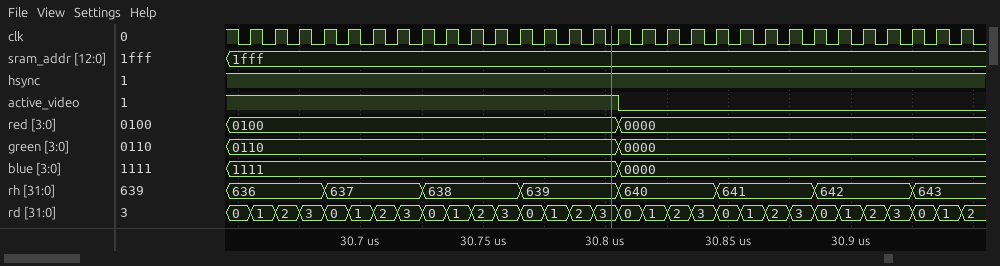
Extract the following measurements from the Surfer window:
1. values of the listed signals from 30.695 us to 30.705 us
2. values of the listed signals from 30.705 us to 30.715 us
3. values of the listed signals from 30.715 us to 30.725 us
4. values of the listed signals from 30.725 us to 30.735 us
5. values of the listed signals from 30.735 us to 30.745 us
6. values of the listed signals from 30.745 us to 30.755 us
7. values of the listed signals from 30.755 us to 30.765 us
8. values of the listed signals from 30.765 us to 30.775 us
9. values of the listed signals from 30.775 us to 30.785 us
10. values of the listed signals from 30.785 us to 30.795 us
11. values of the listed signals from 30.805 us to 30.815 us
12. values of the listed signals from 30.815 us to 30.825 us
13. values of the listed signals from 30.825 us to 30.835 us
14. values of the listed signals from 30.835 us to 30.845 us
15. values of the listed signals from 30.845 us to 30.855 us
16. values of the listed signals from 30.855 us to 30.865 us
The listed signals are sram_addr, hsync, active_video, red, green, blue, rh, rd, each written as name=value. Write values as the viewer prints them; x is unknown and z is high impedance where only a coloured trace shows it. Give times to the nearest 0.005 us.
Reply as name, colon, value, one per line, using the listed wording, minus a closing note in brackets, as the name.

values of the listed signals from 30.695 us to 30.705 us: sram_addr=1fff, hsync=1, active_video=1, red=0100, green=0110, blue=1111, rh=637, rd=1
values of the listed signals from 30.705 us to 30.715 us: sram_addr=1fff, hsync=1, active_video=1, red=0100, green=0110, blue=1111, rh=637, rd=2
values of the listed signals from 30.715 us to 30.725 us: sram_addr=1fff, hsync=1, active_video=1, red=0100, green=0110, blue=1111, rh=637, rd=3
values of the listed signals from 30.725 us to 30.735 us: sram_addr=1fff, hsync=1, active_video=1, red=0100, green=0110, blue=1111, rh=638, rd=0
values of the listed signals from 30.735 us to 30.745 us: sram_addr=1fff, hsync=1, active_video=1, red=0100, green=0110, blue=1111, rh=638, rd=1
values of the listed signals from 30.745 us to 30.755 us: sram_addr=1fff, hsync=1, active_video=1, red=0100, green=0110, blue=1111, rh=638, rd=2
values of the listed signals from 30.755 us to 30.765 us: sram_addr=1fff, hsync=1, active_video=1, red=0100, green=0110, blue=1111, rh=638, rd=3
values of the listed signals from 30.765 us to 30.775 us: sram_addr=1fff, hsync=1, active_video=1, red=0100, green=0110, blue=1111, rh=639, rd=0
values of the listed signals from 30.775 us to 30.785 us: sram_addr=1fff, hsync=1, active_video=1, red=0100, green=0110, blue=1111, rh=639, rd=1
values of the listed signals from 30.785 us to 30.795 us: sram_addr=1fff, hsync=1, active_video=1, red=0100, green=0110, blue=1111, rh=639, rd=2
values of the listed signals from 30.805 us to 30.815 us: sram_addr=1fff, hsync=1, active_video=0, red=0000, green=0000, blue=0000, rh=640, rd=0
values of the listed signals from 30.815 us to 30.825 us: sram_addr=1fff, hsync=1, active_video=0, red=0000, green=0000, blue=0000, rh=640, rd=1
values of the listed signals from 30.825 us to 30.835 us: sram_addr=1fff, hsync=1, active_video=0, red=0000, green=0000, blue=0000, rh=640, rd=2
values of the listed signals from 30.835 us to 30.845 us: sram_addr=1fff, hsync=1, active_video=0, red=0000, green=0000, blue=0000, rh=640, rd=3
values of the listed signals from 30.845 us to 30.855 us: sram_addr=1fff, hsync=1, active_video=0, red=0000, green=0000, blue=0000, rh=641, rd=0
values of the listed signals from 30.855 us to 30.865 us: sram_addr=1fff, hsync=1, active_video=0, red=0000, green=0000, blue=0000, rh=641, rd=1
